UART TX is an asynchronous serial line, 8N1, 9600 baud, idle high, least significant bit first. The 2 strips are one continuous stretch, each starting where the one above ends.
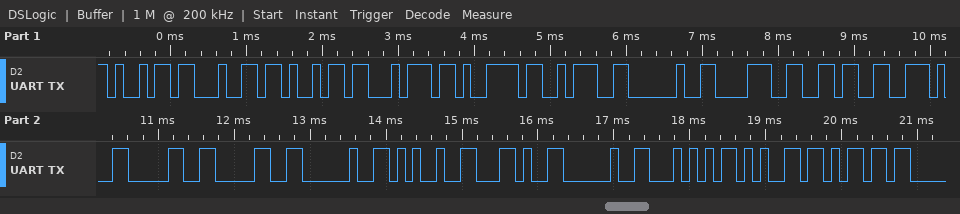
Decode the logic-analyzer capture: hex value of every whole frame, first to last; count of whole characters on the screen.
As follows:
0x69 0x64 0x69 0x74 0x79 0x3A 0x20 0x38 0x36 0x2E 0x30 0x30 0x20 0x25 0x2C 0x20 0x54 0x65 0x6D
19
